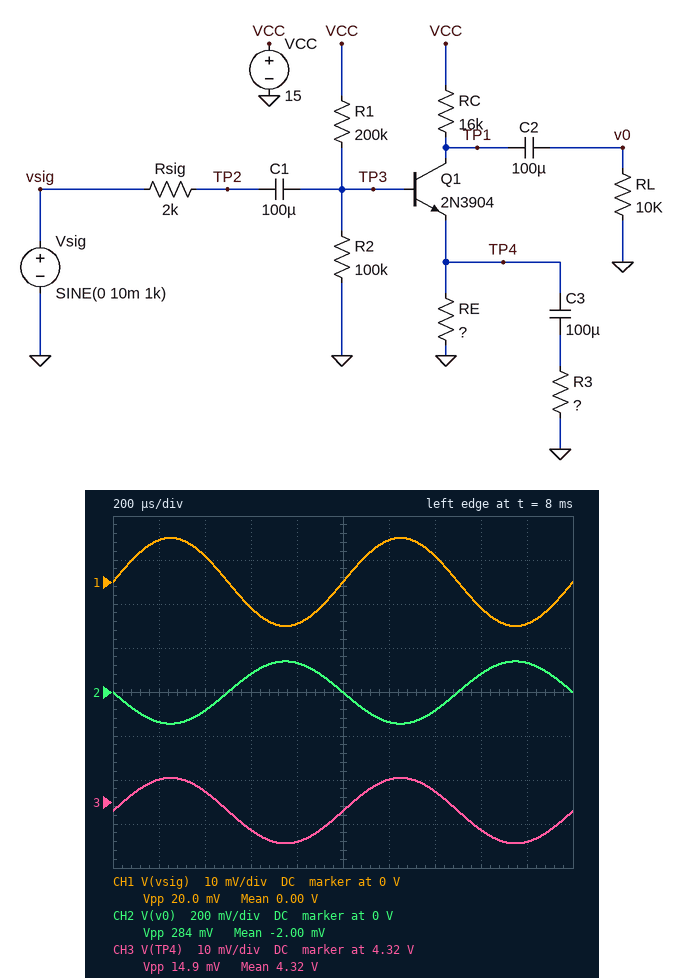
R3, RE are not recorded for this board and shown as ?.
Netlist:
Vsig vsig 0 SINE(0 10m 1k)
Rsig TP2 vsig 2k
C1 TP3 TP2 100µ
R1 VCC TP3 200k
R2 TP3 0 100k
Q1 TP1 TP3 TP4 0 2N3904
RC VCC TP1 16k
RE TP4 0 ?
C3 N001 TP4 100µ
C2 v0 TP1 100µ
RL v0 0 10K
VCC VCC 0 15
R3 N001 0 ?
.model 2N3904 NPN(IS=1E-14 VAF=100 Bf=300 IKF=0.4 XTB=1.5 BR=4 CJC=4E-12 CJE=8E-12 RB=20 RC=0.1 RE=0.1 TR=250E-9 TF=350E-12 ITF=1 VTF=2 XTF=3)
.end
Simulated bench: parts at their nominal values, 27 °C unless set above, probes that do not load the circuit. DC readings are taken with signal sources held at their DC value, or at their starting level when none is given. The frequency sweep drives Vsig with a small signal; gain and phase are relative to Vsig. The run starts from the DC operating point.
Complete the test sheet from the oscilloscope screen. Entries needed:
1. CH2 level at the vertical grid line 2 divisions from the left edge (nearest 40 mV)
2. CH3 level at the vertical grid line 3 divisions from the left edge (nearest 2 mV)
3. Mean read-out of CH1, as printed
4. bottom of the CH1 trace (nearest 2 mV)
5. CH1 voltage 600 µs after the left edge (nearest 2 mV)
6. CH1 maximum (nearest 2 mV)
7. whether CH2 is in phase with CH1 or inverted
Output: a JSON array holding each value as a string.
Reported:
["-80 mV", "4.314 V", "0.00 V", "-10 mV", "-6 mV", "10 mV", "inverted"]
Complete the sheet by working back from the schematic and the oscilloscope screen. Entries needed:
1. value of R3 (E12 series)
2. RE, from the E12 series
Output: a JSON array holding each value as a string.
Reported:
["330 Ω", "15 kΩ"]
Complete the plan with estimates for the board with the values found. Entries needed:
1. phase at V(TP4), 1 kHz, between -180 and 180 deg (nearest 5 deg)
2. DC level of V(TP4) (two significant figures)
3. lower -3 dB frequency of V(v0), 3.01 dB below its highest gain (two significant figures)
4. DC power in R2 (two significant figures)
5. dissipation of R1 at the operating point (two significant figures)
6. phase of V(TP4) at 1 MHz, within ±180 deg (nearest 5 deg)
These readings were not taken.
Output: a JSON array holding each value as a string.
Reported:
["0 deg", "4.3 V", "3.7 Hz", "240 µW", "510 µW", "-20 deg"]
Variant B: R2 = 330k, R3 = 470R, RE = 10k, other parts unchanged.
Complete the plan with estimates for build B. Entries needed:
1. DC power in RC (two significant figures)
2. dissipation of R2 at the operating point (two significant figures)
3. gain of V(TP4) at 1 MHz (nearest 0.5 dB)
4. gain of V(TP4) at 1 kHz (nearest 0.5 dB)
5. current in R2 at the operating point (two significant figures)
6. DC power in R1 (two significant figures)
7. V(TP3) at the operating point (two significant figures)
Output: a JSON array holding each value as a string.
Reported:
["5.1 mW", "130 µW", "-15.5 dB", "-15.0 dB", "20 µA", "360 µW", "6.5 V"]
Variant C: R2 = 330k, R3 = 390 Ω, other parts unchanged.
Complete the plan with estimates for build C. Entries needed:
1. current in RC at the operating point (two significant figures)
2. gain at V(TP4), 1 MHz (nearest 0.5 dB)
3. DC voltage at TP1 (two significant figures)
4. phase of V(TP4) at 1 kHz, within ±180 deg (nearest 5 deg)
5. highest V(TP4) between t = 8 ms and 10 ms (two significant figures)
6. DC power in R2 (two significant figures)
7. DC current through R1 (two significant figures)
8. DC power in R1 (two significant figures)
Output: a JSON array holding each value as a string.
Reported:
["480 µA", "-16.5 dB", "7.4 V", "0 deg", "7.3 V", "190 µW", "35 µA", "250 µW"]
